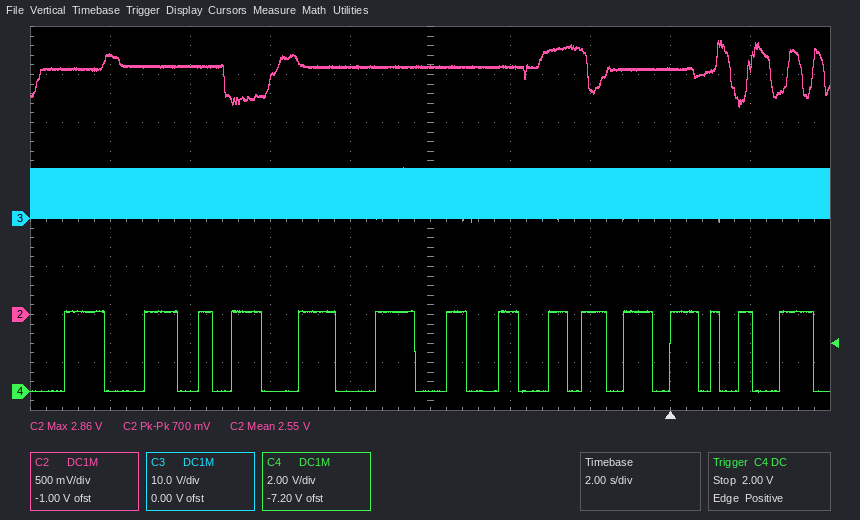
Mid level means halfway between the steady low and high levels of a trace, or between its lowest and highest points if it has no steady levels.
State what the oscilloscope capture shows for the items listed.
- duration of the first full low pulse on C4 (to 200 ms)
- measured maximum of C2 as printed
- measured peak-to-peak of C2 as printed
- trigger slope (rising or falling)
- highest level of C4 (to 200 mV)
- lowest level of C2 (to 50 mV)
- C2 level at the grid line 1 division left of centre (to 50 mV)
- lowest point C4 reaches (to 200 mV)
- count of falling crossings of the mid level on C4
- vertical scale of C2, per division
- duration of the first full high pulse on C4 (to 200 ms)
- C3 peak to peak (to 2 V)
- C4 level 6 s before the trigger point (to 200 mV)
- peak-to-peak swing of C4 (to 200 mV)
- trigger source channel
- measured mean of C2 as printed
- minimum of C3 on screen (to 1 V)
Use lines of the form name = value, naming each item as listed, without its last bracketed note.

duration of the first full low pulse on C4 = 1.0 s
measured maximum of C2 as printed = 2.86 V
measured peak-to-peak of C2 as printed = 700 mV
trigger slope = rising
highest level of C4 = 3.4 V
lowest level of C2 = 2.15 V
C2 level at the grid line 1 division left of centre = 2.55 V
lowest point C4 reaches = 0.0 V
count of falling crossings of the mid level on C4 = 15
vertical scale of C2, per division = 500 mV
duration of the first full high pulse on C4 = 1.0 s
C3 peak to peak = 12 V
C4 level 6 s before the trigger point = 0.0 V
peak-to-peak swing of C4 = 3.4 V
trigger source channel = C4
measured mean of C2 as printed = 2.55 V
minimum of C3 on screen = -1 V
